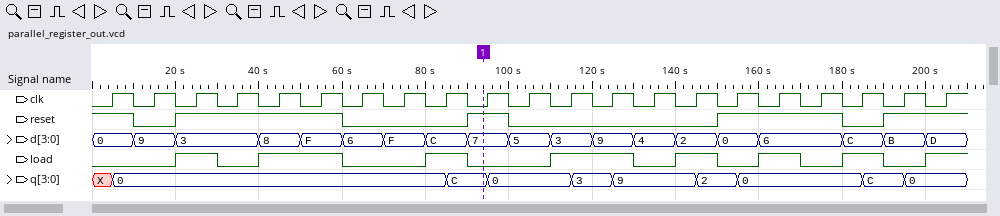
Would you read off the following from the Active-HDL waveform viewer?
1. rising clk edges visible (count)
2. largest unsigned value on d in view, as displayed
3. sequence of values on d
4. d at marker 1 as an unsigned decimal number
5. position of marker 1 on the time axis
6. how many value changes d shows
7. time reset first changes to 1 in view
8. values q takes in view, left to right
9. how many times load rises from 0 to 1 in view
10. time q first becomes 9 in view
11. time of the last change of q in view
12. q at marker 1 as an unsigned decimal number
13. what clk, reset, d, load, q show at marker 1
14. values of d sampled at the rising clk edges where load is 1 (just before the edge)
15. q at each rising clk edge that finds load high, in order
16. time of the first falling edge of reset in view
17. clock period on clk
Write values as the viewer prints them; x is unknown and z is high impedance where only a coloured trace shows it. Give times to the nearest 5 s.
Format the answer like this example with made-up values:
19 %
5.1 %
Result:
21
F
0, 9, 3, 8, F, 6, F, C, 7, 5, 3, 9, 4, 2, 0, 6, C, B, D
7
95 s
18
20 s
X, 0, C, 0, 3, 9, 2, 0, C, 0
8
125 s
195 s
12
clk=0, reset=1, d=7, load=0, q=C
3, 8, F, C, 3, 9, 2, 6, C, D
0, 0, 0, 0, 0, 3, 9, 0, 0, 0
10 s
10 s
